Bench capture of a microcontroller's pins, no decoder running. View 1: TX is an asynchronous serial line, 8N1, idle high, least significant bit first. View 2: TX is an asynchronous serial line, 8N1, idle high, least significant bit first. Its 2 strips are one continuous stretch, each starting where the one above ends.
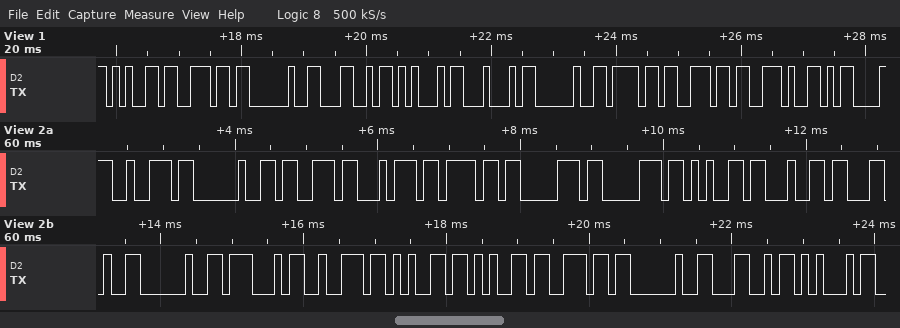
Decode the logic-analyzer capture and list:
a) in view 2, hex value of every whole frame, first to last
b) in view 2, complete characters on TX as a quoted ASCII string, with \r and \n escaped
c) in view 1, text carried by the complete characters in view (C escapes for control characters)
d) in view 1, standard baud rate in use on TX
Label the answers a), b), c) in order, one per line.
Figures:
a) 0x72 0x20 0x73 0x74 0x6F 0x70 0x70 0x65 0x64 0x2C 0x20 0x47 0x72 0x65 0x65 0x6E 0x20 0x4C 0x45
b) "r stopped, Green LE"
c) "en LED on.\r"
d) 9600 baud
